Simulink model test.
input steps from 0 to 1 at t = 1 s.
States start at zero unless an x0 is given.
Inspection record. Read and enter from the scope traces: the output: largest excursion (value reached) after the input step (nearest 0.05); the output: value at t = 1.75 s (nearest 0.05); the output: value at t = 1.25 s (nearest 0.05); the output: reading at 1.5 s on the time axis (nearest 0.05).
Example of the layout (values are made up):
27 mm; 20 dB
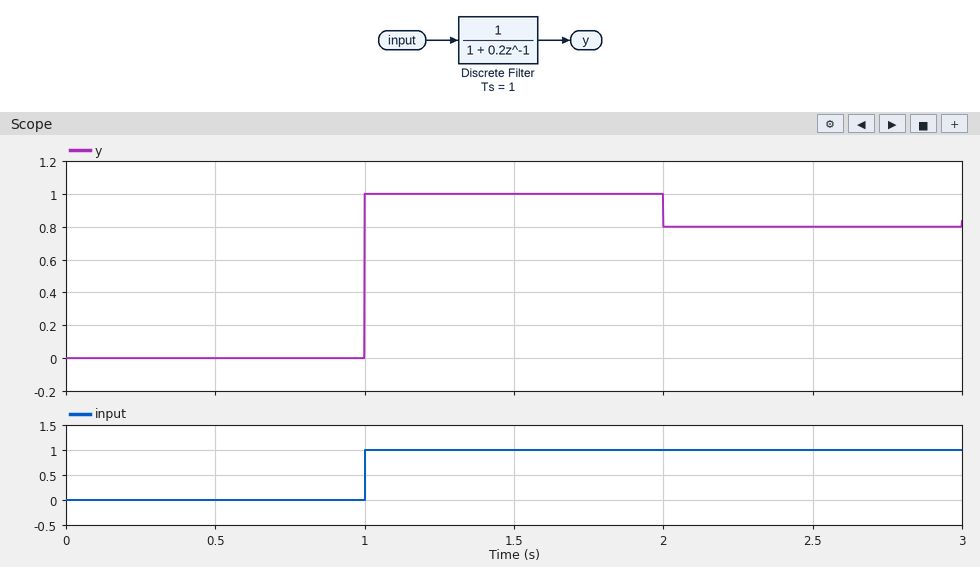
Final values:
1.00; 1.00; 1.00; 1.00
